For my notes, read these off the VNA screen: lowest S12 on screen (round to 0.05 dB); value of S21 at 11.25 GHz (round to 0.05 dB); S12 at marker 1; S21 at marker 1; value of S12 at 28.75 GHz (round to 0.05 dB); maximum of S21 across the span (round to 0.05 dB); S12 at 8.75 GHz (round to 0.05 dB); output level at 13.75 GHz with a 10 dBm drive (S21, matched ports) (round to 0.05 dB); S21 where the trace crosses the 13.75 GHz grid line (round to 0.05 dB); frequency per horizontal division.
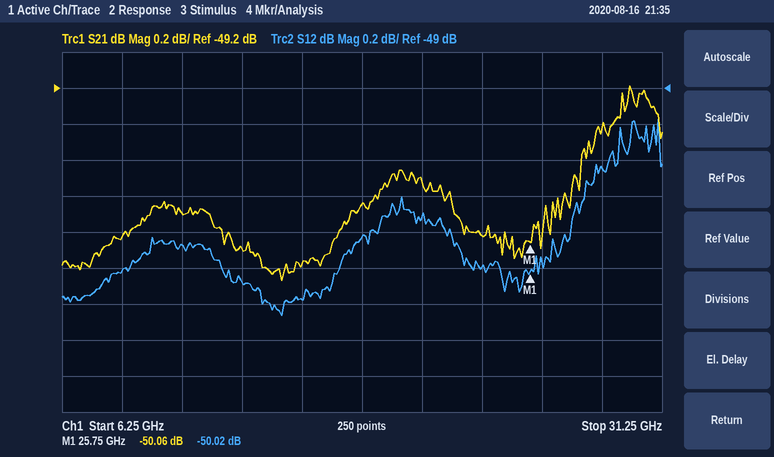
-50.25 dB
-49.90 dB
-50.02 dB
-50.06 dB
-49.45 dB
-49.20 dB
-50.00 dB
-40.10 dBm
-50.10 dB
2.5 GHz
